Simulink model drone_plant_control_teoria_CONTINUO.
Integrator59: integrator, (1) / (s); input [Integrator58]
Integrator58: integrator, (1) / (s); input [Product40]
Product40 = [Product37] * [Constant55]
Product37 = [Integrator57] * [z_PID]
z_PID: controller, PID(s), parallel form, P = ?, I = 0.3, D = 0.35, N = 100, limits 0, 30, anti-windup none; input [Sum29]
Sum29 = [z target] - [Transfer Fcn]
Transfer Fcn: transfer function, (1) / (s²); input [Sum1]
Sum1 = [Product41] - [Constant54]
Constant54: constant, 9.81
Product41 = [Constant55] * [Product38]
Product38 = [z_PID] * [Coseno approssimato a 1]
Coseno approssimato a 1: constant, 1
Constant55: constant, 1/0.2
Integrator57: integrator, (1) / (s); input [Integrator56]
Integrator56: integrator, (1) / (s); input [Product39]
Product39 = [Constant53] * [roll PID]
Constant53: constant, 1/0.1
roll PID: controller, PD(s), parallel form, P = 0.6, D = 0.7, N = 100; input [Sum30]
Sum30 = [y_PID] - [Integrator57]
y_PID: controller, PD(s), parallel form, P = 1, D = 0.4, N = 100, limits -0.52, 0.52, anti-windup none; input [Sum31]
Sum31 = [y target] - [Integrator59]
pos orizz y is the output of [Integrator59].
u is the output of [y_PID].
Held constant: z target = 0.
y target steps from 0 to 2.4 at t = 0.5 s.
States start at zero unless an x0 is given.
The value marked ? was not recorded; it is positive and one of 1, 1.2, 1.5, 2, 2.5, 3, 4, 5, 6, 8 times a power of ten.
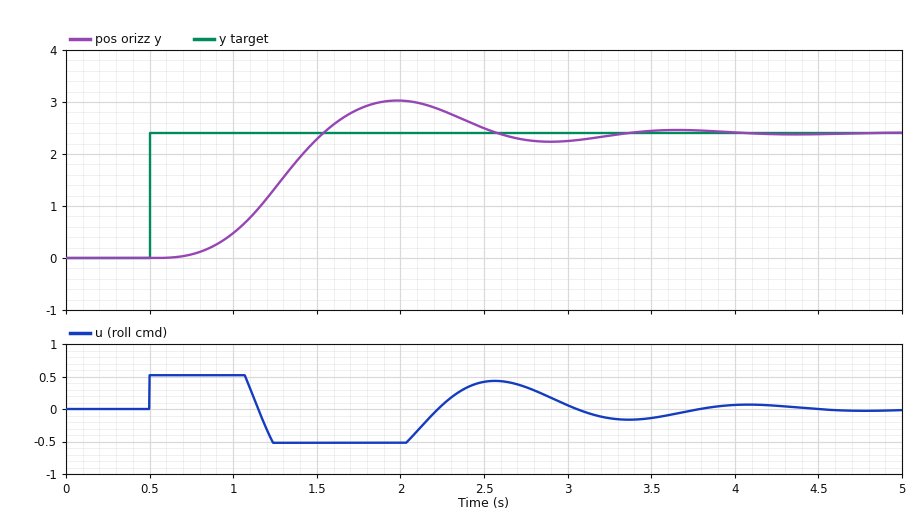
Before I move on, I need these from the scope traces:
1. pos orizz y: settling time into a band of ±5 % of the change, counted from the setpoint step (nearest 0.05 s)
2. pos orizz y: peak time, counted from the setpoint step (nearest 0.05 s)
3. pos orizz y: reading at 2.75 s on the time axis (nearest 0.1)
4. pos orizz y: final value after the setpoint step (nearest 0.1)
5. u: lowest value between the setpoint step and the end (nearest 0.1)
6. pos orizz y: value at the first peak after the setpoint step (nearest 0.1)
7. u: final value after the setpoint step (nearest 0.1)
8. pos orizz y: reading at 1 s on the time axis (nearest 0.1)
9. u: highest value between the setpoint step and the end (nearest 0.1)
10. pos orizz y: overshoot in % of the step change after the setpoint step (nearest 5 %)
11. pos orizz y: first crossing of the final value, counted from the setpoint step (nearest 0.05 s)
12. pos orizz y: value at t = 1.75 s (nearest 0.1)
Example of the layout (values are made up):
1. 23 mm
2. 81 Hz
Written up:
1. 2.60 s
2. 1.50 s
3. 2.3
4. 2.4
5. -0.5
6. 3.0
7. 0.0
8. 0.5
9. 0.5
10. 25 %
11. 1.05 s
12. 2.9
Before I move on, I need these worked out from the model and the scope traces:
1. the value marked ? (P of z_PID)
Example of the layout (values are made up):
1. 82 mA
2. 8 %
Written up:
1. 1
